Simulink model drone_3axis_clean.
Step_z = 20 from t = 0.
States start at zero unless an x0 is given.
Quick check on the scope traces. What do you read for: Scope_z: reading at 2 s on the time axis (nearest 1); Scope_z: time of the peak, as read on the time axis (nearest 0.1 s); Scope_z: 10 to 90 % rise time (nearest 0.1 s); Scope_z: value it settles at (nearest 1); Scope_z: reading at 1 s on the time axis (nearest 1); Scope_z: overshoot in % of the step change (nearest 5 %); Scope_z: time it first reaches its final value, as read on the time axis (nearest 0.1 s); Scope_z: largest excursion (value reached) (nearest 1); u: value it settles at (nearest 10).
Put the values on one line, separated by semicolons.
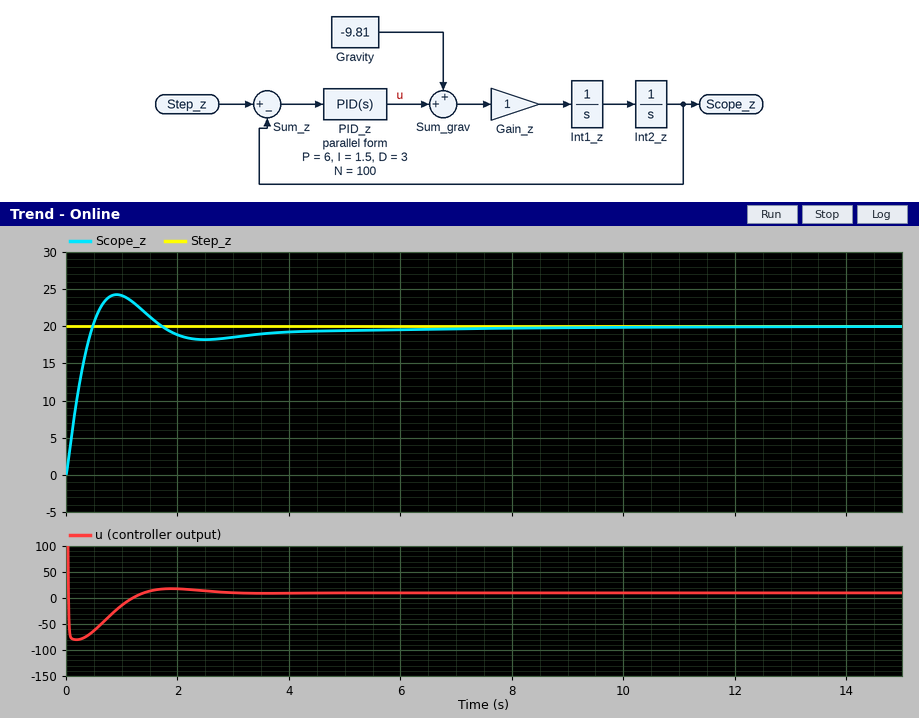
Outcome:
19; 0.9 s; 0.4 s; 20; 24; 20 %; 0.5 s; 24; 10
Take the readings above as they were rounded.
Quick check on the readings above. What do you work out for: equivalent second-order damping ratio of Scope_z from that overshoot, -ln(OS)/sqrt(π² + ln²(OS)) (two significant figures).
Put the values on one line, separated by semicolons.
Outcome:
0.46
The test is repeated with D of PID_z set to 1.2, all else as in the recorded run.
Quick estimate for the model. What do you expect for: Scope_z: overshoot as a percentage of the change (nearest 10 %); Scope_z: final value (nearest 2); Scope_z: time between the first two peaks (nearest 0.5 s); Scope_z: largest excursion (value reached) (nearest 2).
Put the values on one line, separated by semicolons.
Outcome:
50 %; 20; 2.5 s; 30
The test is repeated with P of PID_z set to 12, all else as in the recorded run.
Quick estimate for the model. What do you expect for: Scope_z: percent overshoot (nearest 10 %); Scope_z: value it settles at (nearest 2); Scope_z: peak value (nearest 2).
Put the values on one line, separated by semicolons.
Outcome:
30 %; 20; 26
